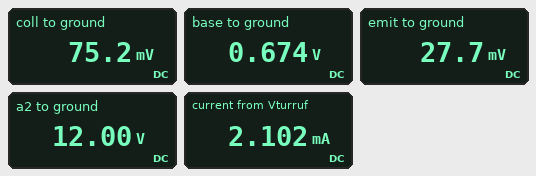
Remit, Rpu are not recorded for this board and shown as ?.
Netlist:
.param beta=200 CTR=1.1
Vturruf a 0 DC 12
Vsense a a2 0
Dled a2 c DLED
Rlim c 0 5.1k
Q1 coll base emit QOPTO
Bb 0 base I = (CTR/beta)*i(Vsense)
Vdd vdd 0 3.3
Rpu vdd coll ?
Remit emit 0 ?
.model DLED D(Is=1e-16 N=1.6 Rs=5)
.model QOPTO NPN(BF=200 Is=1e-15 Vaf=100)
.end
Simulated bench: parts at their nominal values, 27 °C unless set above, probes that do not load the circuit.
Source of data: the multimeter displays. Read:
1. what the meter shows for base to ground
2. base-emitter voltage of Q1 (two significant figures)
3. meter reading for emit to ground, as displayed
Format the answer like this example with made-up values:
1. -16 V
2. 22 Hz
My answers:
1. 0.674 V
2. 650 mV
3. 27.7 mV
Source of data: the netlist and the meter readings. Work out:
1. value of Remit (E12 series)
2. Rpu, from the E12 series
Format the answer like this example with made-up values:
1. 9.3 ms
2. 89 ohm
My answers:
1. 470 Ω
2. 68 kΩ
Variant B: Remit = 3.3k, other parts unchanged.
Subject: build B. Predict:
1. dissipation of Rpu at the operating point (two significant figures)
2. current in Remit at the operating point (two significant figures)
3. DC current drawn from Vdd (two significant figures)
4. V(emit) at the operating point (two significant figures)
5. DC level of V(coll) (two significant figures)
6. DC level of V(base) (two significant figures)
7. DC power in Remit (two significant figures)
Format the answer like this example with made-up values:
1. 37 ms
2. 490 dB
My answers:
1. 140 µW
2. 57 µA
3. 45 µA
4. 190 mV
5. 230 mV
6. 830 mV
7. 11 µW
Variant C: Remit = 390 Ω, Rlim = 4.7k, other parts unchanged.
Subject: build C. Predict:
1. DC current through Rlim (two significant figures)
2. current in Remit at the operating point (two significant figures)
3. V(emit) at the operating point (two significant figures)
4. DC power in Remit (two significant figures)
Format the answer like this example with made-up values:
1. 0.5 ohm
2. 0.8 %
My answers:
1. 2.3 mA
2. 60 µA
3. 23 mV
4. 1.4 µW
